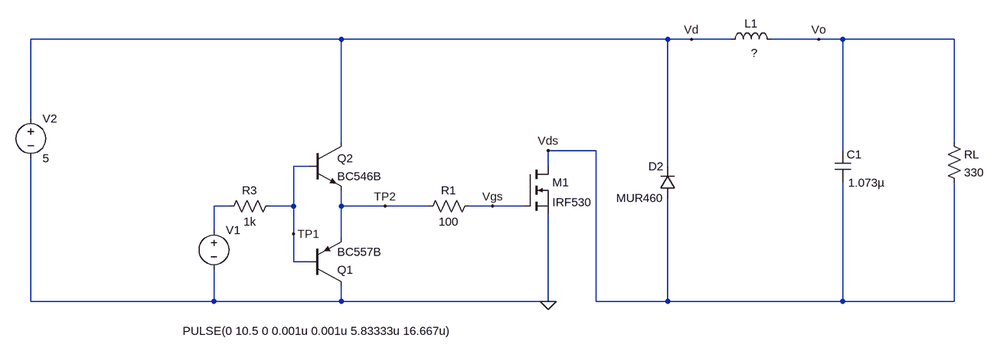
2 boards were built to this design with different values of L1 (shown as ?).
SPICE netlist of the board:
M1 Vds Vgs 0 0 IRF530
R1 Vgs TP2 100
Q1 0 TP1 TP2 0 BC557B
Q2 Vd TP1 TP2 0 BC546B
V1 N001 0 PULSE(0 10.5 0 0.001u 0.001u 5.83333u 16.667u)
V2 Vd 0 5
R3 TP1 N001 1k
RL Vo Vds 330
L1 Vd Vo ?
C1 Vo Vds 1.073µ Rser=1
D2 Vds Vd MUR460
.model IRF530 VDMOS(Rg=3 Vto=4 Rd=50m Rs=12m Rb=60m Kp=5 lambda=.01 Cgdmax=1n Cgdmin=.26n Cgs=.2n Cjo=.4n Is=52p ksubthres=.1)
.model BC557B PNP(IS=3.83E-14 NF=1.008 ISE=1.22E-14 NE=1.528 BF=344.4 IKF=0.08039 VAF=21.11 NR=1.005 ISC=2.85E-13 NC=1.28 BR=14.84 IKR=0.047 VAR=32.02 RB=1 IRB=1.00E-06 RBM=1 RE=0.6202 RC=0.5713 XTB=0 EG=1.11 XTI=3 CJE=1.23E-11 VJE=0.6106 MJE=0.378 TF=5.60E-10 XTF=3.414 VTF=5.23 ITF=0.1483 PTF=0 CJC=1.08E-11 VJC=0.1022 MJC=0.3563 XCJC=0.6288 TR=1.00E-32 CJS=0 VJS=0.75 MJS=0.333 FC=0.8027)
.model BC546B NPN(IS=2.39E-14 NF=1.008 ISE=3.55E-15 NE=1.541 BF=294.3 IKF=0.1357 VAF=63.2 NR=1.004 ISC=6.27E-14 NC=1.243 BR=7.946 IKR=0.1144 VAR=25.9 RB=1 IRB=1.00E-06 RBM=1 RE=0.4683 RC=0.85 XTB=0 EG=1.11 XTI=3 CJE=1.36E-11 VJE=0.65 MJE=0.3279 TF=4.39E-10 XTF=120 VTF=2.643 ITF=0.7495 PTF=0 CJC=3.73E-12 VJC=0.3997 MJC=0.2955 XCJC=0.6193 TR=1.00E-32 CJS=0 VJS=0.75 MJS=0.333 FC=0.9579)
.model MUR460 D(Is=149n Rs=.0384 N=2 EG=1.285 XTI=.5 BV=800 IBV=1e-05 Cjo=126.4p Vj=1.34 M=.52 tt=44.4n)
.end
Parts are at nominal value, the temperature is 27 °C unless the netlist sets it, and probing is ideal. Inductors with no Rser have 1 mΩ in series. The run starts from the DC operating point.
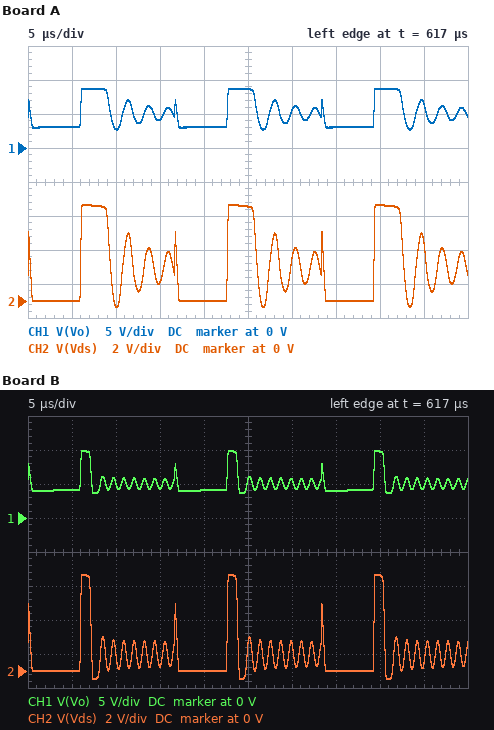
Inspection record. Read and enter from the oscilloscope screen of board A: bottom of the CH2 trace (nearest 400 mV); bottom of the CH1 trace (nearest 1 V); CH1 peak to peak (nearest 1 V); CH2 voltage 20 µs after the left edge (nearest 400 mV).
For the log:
-400 mV
3 V
6 V
0 V
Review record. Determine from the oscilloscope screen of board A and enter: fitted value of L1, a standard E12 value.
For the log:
270 µH
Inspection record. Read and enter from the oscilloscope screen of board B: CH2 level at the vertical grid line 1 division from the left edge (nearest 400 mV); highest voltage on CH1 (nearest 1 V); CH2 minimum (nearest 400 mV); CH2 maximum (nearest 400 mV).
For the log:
0 V
10 V
-400 mV
5.6 V
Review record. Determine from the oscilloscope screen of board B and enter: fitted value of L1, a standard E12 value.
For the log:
68 µH
